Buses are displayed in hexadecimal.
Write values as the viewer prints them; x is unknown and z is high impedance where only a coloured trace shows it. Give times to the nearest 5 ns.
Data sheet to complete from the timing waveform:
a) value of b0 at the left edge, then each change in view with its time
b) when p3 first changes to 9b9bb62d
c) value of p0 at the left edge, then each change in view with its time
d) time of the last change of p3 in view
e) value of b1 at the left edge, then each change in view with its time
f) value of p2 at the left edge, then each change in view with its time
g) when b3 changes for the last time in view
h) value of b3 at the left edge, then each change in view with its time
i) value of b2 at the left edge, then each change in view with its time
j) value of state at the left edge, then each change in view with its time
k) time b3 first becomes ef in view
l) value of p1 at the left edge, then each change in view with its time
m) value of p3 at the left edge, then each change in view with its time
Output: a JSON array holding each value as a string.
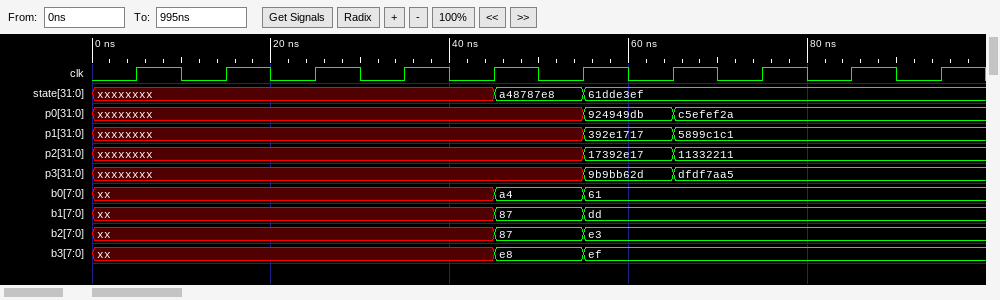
["xx, a4 at 45 ns, 61 at 55 ns", "55 ns", "xxxxxxxx, 924949db at 55 ns, c5efef2a at 65 ns", "65 ns", "xx, 87 at 45 ns, dd at 55 ns", "xxxxxxxx, 17392e17 at 55 ns, 11332211 at 65 ns", "55 ns", "xx, e8 at 45 ns, ef at 55 ns", "xx, 87 at 45 ns, e3 at 55 ns", "xxxxxxxx, a48787e8 at 45 ns, 61dde3ef at 55 ns", "55 ns", "xxxxxxxx, 392e1717 at 55 ns, 5899c1c1 at 65 ns", "xxxxxxxx, 9b9bb62d at 55 ns, dfdf7aa5 at 65 ns"]
